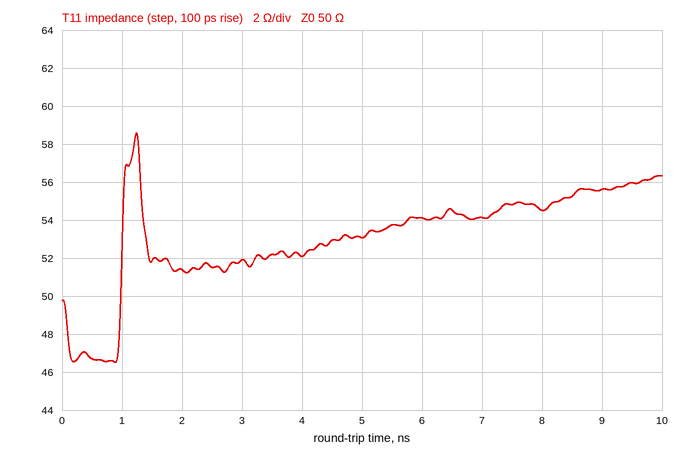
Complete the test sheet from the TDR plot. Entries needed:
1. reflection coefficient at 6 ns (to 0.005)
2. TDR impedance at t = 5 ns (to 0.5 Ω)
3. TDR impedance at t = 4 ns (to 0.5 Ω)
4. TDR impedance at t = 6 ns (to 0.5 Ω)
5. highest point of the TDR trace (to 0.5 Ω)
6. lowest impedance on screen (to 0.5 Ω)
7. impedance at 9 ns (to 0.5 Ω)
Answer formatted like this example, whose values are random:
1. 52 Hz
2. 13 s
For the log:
1. +0.040
2. 53.0 Ω
3. 52.0 Ω
4. 54.0 Ω
5. 58.5 Ω
6. 46.5 Ω
7. 55.5 Ω
